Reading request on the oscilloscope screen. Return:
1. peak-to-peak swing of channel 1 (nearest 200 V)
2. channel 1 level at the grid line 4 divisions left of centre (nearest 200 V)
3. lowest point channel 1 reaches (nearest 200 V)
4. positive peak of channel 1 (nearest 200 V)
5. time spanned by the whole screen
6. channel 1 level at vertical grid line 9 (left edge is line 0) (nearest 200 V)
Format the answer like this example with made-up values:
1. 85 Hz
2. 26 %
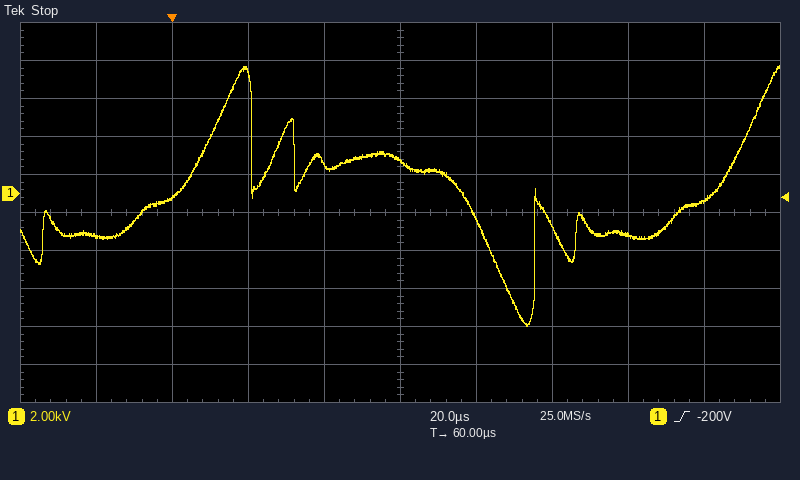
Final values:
1. 13.8 kV
2. -2.2 kV
3. -7.0 kV
4. 6.8 kV
5. 200 µs
6. -400 V
